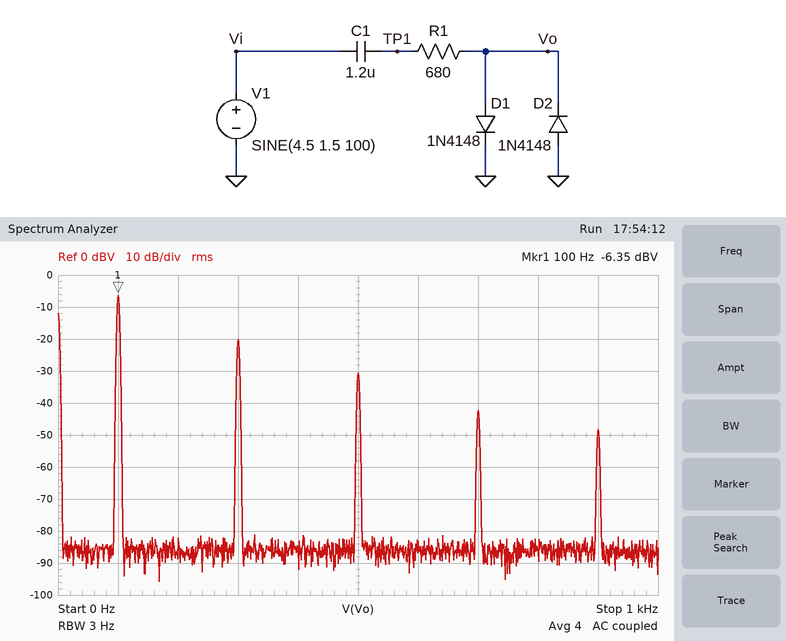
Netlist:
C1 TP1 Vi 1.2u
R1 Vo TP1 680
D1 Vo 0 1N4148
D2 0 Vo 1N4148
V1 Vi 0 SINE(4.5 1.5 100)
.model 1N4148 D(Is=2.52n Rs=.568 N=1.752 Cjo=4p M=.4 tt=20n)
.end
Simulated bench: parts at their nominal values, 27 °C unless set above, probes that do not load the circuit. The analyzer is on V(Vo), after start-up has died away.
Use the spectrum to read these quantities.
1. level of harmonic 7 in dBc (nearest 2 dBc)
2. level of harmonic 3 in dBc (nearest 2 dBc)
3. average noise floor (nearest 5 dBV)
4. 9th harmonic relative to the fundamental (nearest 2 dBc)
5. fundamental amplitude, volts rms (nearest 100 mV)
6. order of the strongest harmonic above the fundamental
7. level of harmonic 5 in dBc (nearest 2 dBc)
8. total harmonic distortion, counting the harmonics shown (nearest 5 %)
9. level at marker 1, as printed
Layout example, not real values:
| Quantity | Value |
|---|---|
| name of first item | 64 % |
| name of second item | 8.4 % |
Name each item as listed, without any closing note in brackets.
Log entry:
| Quantity | Value |
|---|---|
| level of harmonic 7 in dBc | -36 dBc |
| level of harmonic 3 in dBc | -14 dBc |
| average noise floor | -85 dBV |
| 9th harmonic relative to the fundamental | -42 dBc |
| fundamental amplitude, volts rms | 500 mV |
| order of the strongest harmonic above the fundamental | 3 |
| level of harmonic 5 in dBc | -24 dBc |
| total harmonic distortion, counting the harmonics shown | 20 % |
| level at marker 1, as printed | -6.35 dBV |
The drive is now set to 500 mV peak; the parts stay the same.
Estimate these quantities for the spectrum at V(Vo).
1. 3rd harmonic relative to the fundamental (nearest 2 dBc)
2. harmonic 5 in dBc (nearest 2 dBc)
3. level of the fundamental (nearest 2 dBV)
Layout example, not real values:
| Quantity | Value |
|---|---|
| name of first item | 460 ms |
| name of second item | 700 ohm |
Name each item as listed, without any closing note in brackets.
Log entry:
| Quantity | Value |
|---|---|
| 3rd harmonic relative to the fundamental | -30 dBc |
| harmonic 5 in dBc | -40 dBc |
| level of the fundamental | -10 dBV |
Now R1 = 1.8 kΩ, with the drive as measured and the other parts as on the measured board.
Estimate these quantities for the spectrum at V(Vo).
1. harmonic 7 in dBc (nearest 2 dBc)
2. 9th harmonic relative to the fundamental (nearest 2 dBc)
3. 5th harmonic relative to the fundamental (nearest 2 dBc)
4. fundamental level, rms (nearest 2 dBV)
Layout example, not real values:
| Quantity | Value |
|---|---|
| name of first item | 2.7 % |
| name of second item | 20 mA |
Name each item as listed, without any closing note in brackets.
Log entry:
| Quantity | Value |
|---|---|
| harmonic 7 in dBc | -30 dBc |
| 9th harmonic relative to the fundamental | -44 dBc |
| 5th harmonic relative to the fundamental | -22 dBc |
| fundamental level, rms | -6 dBV |
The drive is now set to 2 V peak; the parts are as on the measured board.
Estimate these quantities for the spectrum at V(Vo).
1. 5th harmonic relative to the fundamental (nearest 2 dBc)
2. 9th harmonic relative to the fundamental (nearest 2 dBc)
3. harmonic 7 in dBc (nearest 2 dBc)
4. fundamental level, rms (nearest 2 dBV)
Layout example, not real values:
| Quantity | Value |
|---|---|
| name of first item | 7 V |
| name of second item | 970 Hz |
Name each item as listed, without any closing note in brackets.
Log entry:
| Quantity | Value |
|---|---|
| 5th harmonic relative to the fundamental | -22 dBc |
| 9th harmonic relative to the fundamental | -40 dBc |
| harmonic 7 in dBc | -30 dBc |
| fundamental level, rms | -6 dBV |
